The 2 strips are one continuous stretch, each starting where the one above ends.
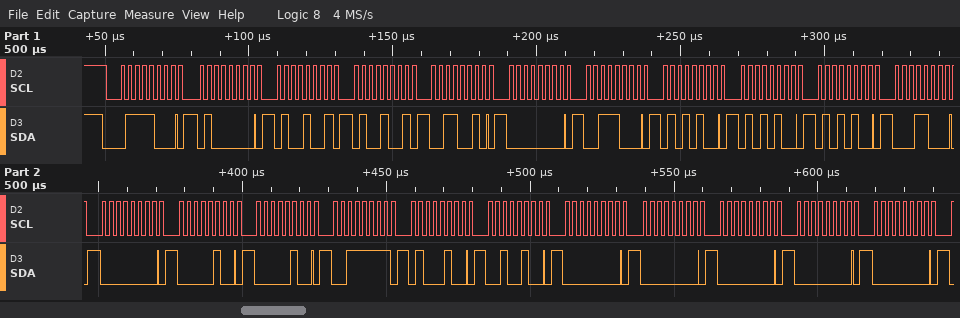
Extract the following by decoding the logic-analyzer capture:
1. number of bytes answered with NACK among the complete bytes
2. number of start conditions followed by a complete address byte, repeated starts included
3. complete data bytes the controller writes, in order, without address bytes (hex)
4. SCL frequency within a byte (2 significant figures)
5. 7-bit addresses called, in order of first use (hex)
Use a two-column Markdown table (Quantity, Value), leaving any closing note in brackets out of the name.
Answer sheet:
| Quantity | Value |
|---|---|
| number of bytes answered with NACK among the complete bytes | 0 |
| number of start conditions followed by a complete address byte, repeated starts included | 1 |
| complete data bytes the controller writes, in order, without address bytes | 40 49 49 32 00 38 54 54 54 18 00 04 04 3F 44 24 00 00 00 00 00 |
| SCL frequency within a byte | 400 kHz |
| 7-bit addresses called, in order of first use | 0x3C |
